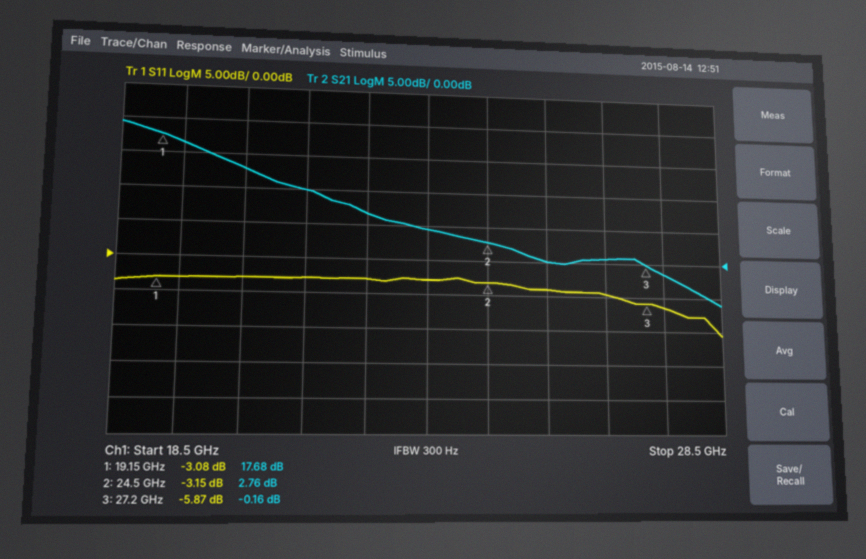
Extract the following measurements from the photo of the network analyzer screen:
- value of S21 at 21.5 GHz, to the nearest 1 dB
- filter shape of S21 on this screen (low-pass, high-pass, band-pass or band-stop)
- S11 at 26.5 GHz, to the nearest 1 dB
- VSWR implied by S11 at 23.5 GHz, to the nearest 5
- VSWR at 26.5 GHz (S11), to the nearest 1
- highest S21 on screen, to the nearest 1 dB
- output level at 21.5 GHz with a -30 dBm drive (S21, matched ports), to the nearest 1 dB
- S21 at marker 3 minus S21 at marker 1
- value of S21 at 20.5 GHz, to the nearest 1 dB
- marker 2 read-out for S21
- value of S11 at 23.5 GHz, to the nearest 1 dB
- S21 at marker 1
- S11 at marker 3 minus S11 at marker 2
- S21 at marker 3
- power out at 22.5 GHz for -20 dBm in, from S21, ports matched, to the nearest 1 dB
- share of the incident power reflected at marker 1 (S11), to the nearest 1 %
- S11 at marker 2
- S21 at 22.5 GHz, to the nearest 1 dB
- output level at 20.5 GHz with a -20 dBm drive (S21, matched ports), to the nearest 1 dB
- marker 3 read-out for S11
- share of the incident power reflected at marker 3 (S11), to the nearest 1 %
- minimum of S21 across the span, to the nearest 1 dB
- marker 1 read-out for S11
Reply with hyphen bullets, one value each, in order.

- 10 dB
- low-pass
- -5 dB
- 5
- 4
- 19 dB
- -20 dBm
- -17.84 dB
- 13 dB
- 2.76 dB
- -3 dB
- 17.68 dB
- -2.72 dB
- -0.16 dB
- -13 dBm
- 49 %
- -3.15 dB
- 7 dB
- -7 dBm
- -5.87 dB
- 26 %
- -6 dB
- -3.08 dB
